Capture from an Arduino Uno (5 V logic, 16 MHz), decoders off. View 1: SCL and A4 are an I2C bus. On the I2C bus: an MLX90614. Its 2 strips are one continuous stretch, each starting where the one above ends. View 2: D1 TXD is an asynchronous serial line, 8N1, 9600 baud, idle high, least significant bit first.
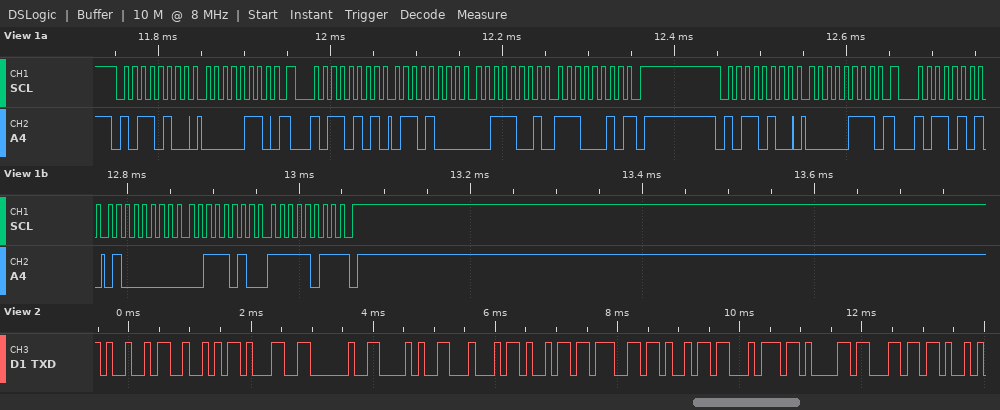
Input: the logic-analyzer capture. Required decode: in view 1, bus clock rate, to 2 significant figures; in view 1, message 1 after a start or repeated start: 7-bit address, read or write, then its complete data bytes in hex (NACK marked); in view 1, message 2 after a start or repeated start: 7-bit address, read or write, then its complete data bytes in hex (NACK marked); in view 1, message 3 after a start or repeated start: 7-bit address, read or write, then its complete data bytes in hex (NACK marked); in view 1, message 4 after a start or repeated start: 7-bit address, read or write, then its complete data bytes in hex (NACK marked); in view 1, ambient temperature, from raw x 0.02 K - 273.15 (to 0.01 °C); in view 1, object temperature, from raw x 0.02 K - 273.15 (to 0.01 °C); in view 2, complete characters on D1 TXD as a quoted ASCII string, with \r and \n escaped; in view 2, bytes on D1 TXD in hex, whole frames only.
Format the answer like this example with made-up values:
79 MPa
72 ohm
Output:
100 kHz
0x5A write: 06
0x5A read: 68 39 E2 NACK
0x5A write: 07
0x5A read: 40 3A FB NACK
20.77 °C
25.09 °C
"IR1 (Digital"
49 52 31 20 28 44 69 67 69 74 61 6C
